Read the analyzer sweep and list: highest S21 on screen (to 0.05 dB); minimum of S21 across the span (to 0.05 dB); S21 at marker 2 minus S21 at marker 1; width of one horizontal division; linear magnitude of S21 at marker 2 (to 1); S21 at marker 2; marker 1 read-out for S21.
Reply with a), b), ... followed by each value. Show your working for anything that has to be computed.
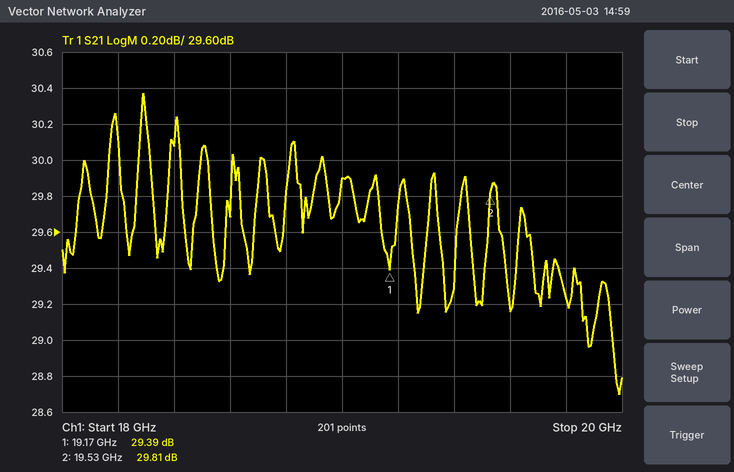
a) 30.35 dB
b) 28.70 dB
c) 29.81 − (29.39) = 0.42 dB
d) 200 MHz
e) 10^(29.81/20) ≈ 31
f) 29.81 dB
g) 29.39 dB
